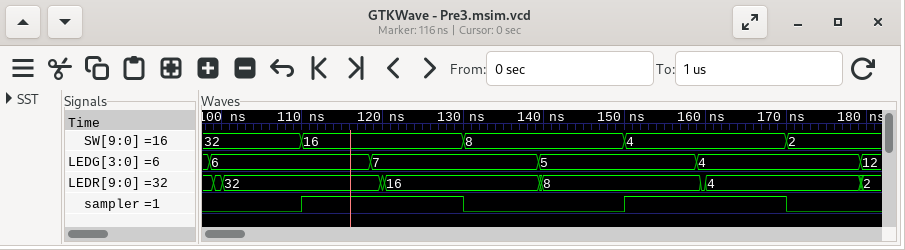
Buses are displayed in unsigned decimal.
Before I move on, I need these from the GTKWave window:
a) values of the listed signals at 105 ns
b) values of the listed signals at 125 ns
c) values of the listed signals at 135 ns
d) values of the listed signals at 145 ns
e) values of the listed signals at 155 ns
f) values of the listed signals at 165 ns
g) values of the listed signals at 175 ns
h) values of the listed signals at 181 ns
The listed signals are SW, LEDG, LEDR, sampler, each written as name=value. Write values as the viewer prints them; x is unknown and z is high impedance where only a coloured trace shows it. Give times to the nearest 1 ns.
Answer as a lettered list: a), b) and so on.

a) SW=32, LEDG=6, LEDR=32, sampler=0
b) SW=16, LEDG=7, LEDR=16, sampler=1
c) SW=8, LEDG=7, LEDR=16, sampler=0
d) SW=8, LEDG=5, LEDR=8, sampler=0
e) SW=4, LEDG=5, LEDR=8, sampler=1
f) SW=4, LEDG=4, LEDR=4, sampler=1
g) SW=2, LEDG=4, LEDR=4, sampler=0
h) SW=2, LEDG=12, LEDR=2, sampler=0
